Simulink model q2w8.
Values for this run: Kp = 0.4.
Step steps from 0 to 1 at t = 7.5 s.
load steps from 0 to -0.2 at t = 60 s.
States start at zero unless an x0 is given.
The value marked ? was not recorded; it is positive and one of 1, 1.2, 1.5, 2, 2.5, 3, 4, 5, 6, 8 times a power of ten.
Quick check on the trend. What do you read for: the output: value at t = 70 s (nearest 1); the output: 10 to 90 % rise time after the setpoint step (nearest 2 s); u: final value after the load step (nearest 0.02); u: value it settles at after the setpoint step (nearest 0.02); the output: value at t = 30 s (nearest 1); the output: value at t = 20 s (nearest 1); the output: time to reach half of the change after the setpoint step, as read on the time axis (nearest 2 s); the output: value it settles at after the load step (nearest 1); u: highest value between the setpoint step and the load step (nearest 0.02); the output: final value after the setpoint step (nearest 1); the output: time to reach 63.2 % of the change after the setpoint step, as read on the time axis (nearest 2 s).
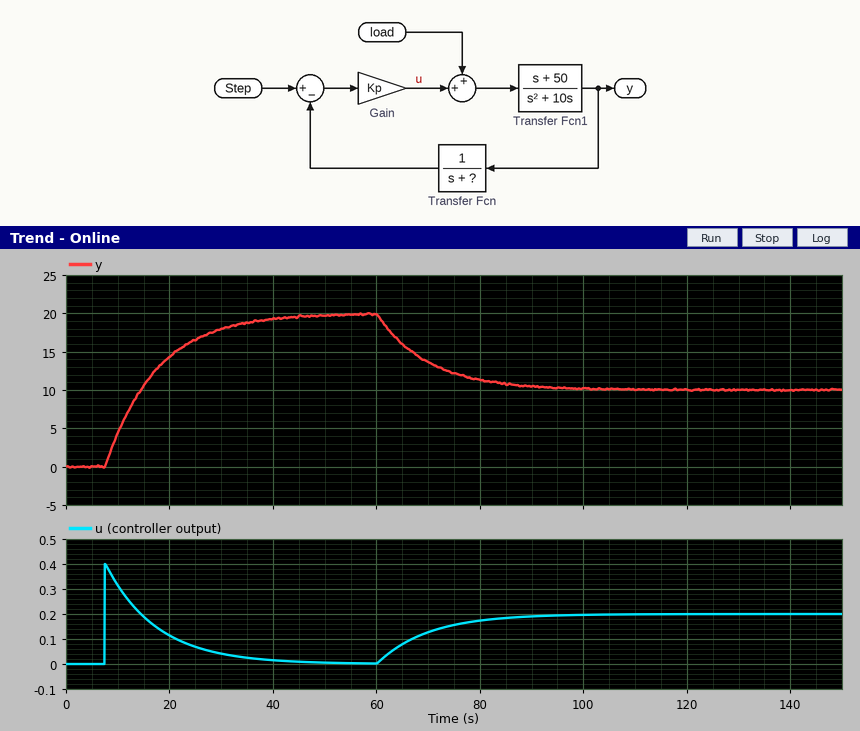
14
22 s
0.20
0.00
18
14
14 s
10
0.40
20
18 s
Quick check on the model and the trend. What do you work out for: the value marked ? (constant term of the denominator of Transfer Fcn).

20
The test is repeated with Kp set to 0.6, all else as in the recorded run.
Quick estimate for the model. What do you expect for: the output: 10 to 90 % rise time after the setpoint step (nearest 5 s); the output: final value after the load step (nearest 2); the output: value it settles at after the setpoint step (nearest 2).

15 s
14
20
